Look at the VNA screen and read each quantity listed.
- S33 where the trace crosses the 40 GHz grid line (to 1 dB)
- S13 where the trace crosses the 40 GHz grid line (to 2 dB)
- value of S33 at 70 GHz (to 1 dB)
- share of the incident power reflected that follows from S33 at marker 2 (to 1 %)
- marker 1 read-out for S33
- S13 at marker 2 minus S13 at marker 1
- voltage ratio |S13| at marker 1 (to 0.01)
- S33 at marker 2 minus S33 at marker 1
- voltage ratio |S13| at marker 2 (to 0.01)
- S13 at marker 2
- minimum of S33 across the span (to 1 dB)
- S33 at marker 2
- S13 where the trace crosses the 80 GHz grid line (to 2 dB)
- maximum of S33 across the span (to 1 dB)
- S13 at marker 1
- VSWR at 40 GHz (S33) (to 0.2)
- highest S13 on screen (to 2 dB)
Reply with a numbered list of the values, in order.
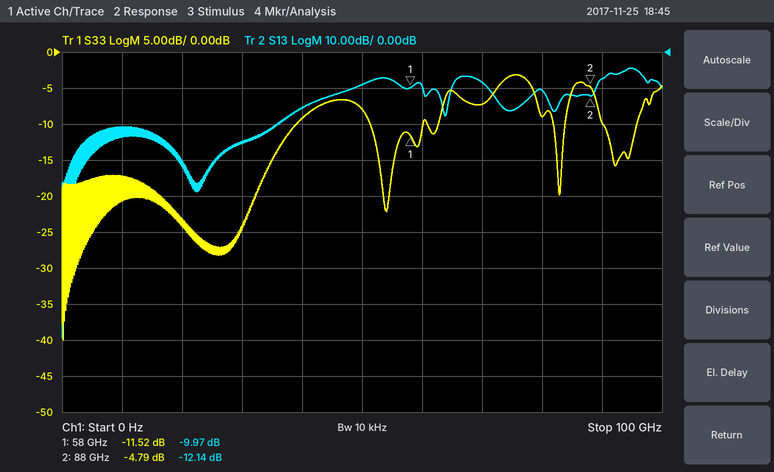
1. -9 dB
2. -16 dB
3. -7 dB
4. 33 %
5. -11.52 dB
6. -2.17 dB
7. 0.32
8. 6.73 dB
9. 0.25
10. -12.14 dB
11. -40 dB
12. -4.79 dB
13. -10 dB
14. -3 dB
15. -9.97 dB
16. 2.0
17. -4 dB
